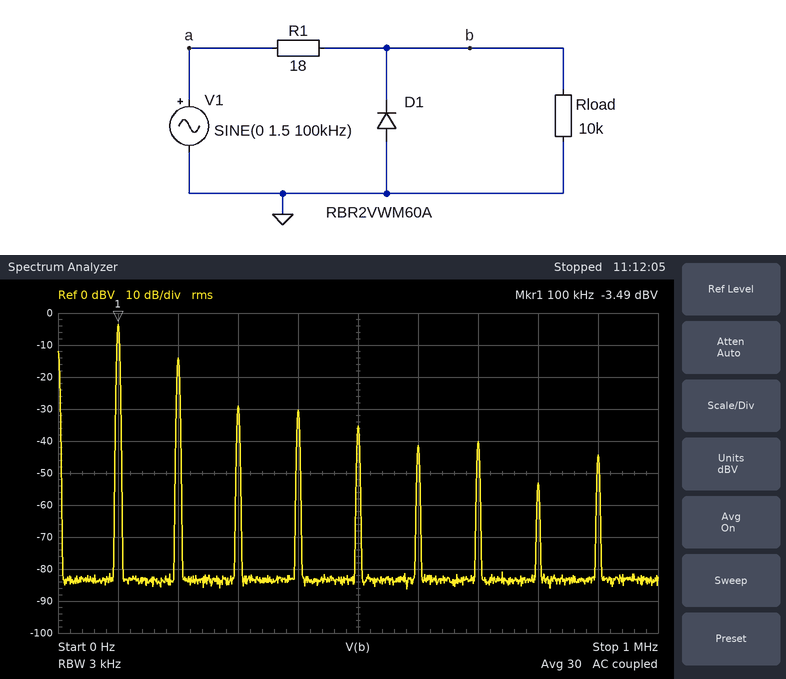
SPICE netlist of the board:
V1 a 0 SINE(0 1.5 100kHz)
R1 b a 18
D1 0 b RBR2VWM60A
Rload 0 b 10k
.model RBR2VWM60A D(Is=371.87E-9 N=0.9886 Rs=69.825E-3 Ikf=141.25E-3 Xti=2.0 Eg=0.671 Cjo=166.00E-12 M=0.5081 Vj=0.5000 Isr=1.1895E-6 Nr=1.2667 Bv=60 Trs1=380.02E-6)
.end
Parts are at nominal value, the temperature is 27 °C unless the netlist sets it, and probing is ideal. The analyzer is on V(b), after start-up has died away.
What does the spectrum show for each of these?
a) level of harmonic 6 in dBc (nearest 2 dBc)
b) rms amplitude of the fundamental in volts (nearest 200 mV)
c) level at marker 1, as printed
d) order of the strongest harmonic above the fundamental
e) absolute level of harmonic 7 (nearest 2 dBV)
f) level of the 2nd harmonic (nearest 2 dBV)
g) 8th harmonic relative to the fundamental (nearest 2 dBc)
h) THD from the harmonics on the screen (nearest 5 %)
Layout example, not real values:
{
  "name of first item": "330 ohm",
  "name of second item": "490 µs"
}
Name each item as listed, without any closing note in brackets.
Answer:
{
  "level of harmonic 6 in dBc": "-38 dBc",
  "rms amplitude of the fundamental in volts": "600 mV",
  "level at marker 1, as printed": "-3.49 dBV",
  "order of the strongest harmonic above the fundamental": "2",
  "absolute level of harmonic 7": "-40 dBV",
  "level of the 2nd harmonic": "-14 dBV",
  "8th harmonic relative to the fundamental": "-50 dBc",
  "THD from the harmonics on the screen": "30 %"
}
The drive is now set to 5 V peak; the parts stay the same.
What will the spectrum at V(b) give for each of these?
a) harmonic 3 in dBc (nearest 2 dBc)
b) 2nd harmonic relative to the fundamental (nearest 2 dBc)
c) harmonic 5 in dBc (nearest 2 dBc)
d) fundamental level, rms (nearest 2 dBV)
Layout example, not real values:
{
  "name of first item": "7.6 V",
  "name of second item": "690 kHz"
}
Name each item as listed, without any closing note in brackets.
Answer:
{
  "harmonic 3 in dBc": "-32 dBc",
  "2nd harmonic relative to the fundamental": "-8 dBc",
  "harmonic 5 in dBc": "-38 dBc",
  "fundamental level, rms": "6 dBV"
}
